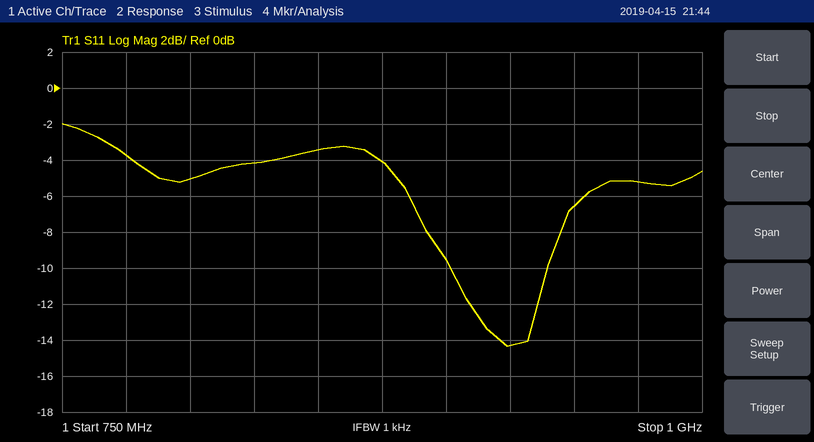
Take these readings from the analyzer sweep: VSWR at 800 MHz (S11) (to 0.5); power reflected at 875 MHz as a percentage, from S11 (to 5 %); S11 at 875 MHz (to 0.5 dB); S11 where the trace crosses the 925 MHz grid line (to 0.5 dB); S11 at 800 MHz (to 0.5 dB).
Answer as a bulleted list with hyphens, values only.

- 3.5
- 40 %
- -4.0 dB
- -14.5 dB
- -5.0 dB
